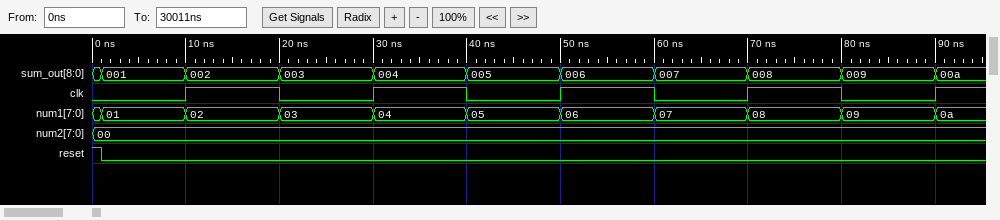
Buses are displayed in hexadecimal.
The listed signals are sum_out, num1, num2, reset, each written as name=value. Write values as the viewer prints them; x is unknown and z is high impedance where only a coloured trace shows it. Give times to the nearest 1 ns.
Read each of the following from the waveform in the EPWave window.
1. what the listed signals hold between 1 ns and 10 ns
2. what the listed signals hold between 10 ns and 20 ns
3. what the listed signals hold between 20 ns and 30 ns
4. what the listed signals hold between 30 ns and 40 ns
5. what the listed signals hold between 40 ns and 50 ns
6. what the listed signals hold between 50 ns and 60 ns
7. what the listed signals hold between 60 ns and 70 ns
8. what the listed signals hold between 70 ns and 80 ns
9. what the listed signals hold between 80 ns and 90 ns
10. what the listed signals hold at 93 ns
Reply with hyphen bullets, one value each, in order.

- sum_out=001, num1=01, num2=00, reset=0
- sum_out=002, num1=02, num2=00, reset=0
- sum_out=003, num1=03, num2=00, reset=0
- sum_out=004, num1=04, num2=00, reset=0
- sum_out=005, num1=05, num2=00, reset=0
- sum_out=006, num1=06, num2=00, reset=0
- sum_out=007, num1=07, num2=00, reset=0
- sum_out=008, num1=08, num2=00, reset=0
- sum_out=009, num1=09, num2=00, reset=0
- sum_out=00a, num1=0a, num2=00, reset=0
